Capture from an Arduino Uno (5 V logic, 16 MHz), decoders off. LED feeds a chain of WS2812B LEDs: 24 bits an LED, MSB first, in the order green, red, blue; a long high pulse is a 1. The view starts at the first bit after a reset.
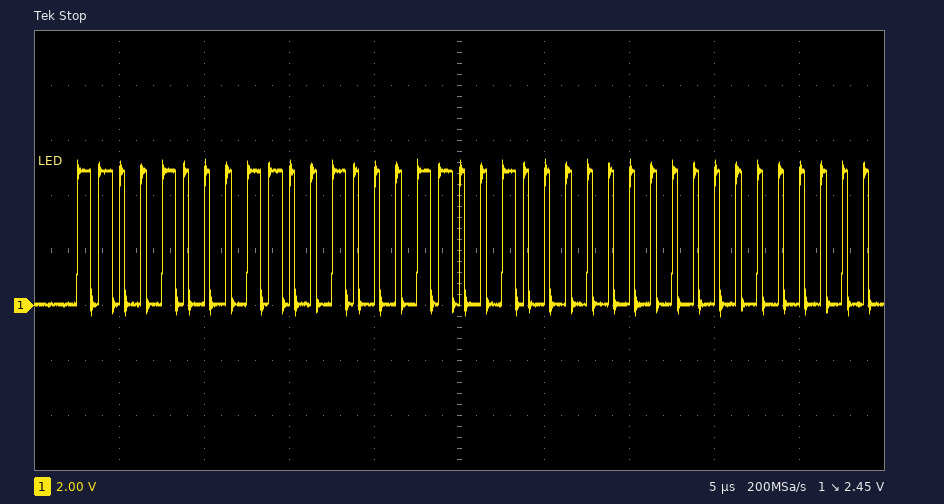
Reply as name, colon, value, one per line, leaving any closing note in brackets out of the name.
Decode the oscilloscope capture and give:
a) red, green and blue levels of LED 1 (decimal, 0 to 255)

red, green and blue levels of LED 1: 200, 200, 200
